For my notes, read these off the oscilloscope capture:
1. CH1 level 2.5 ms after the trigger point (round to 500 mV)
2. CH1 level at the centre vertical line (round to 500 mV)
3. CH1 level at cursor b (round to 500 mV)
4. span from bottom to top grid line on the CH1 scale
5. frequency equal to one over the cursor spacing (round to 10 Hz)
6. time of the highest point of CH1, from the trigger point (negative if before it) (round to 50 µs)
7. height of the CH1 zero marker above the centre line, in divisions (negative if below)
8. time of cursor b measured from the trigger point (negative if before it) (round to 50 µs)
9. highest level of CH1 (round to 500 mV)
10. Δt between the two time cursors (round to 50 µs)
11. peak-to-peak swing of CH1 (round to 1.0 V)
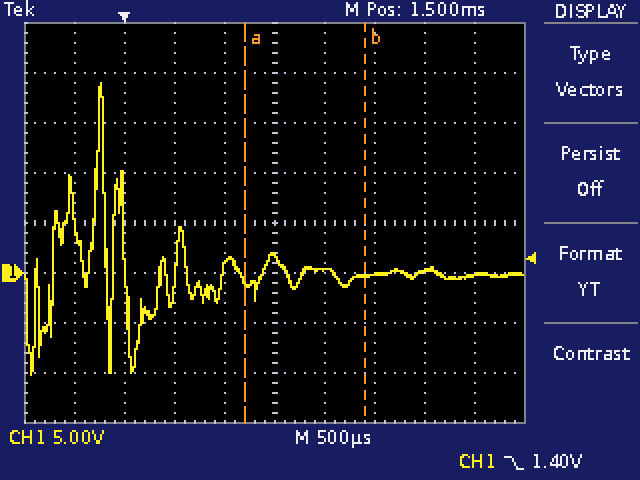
0.0 V
1.5 V
-500 mV
40 V
830 Hz
-250 µs
-1.0 div
+2.40 ms
19.0 V
1.20 ms
29.0 V
